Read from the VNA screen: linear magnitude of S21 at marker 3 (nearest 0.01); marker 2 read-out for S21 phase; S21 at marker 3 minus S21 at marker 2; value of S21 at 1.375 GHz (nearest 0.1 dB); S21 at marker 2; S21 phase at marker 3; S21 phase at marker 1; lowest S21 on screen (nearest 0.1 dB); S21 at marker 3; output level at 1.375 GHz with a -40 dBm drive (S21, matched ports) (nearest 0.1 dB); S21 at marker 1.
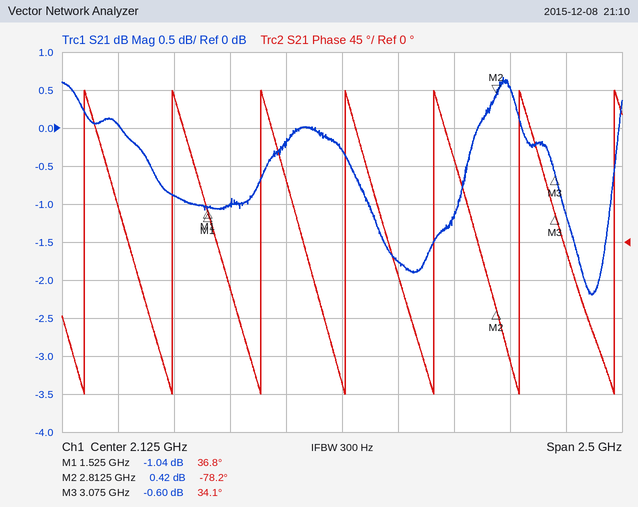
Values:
0.93
-78.2°
-1.02 dB
-0.9 dB
0.42 dB
34.1°
36.8°
-2.2 dB
-0.60 dB
-40.9 dBm
-1.04 dB
